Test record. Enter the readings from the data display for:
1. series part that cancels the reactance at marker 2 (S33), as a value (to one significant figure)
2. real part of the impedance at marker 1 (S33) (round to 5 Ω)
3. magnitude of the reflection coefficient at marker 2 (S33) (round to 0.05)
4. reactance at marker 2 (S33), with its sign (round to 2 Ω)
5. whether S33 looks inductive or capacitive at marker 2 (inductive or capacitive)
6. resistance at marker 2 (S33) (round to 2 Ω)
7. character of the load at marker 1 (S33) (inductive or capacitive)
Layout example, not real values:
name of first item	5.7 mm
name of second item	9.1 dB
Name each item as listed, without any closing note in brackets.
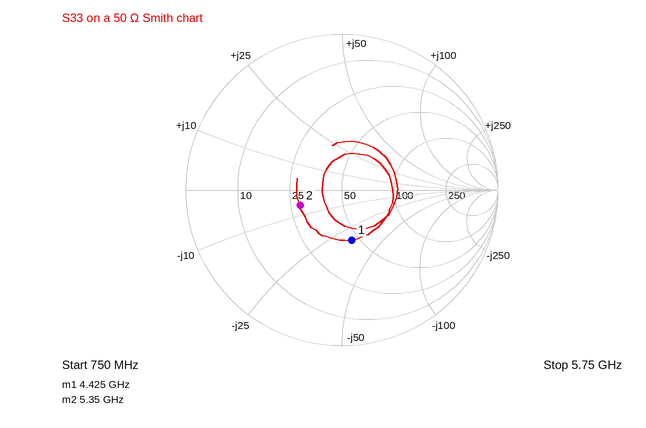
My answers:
series part that cancels the reactance at marker 2 (S33), as a value	200 pH
real part of the impedance at marker 1 (S33)	45 Ω
magnitude of the reflection coefficient at marker 2 (S33)	0.30
reactance at marker 2 (S33), with its sign	-6 Ω
whether S33 looks inductive or capacitive at marker 2	capacitive
resistance at marker 2 (S33)	28 Ω
character of the load at marker 1 (S33)	capacitive
